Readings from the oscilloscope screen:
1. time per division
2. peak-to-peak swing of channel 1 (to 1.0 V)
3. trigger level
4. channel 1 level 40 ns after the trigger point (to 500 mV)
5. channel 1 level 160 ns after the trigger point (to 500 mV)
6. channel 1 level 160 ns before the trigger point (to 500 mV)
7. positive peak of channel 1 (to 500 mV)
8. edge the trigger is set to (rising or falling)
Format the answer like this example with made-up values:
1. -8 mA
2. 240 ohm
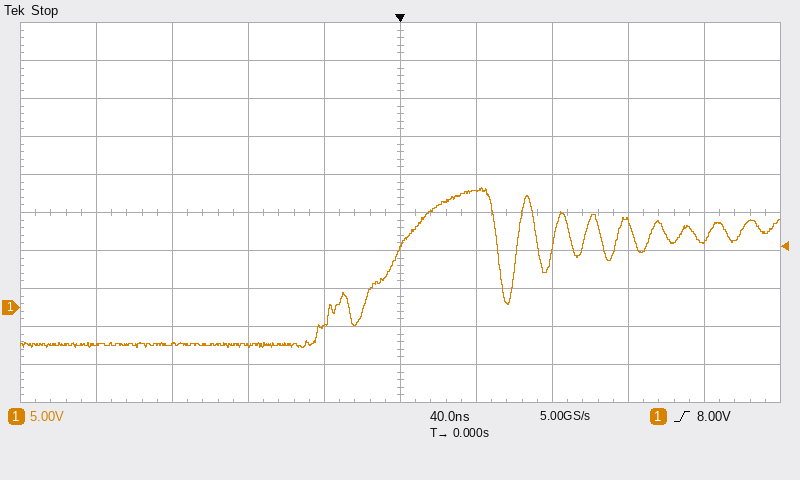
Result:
1. 40 ns
2. 21.0 V
3. 8.00 V
4. 15.5 V
5. 9.0 V
6. -5.0 V
7. 16.0 V
8. rising
